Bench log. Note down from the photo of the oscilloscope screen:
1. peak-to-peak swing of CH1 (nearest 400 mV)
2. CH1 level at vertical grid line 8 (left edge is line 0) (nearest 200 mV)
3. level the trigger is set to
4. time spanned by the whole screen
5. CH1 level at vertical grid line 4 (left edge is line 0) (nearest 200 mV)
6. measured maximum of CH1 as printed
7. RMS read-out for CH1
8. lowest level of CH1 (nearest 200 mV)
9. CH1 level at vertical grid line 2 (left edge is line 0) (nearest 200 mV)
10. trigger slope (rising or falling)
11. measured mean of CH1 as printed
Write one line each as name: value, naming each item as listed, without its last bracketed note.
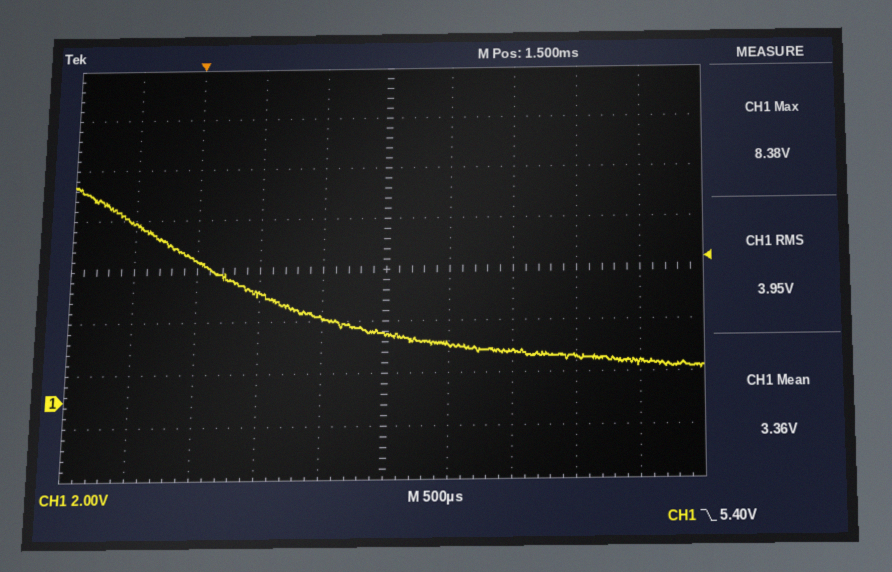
peak-to-peak swing of CH1: 7.2 V
CH1 level at vertical grid line 8 (left edge is line 0): 1.6 V
level the trigger is set to: 5.40 V
time spanned by the whole screen: 5 ms
CH1 level at vertical grid line 4 (left edge is line 0): 3.2 V
measured maximum of CH1 as printed: 8.38 V
RMS read-out for CH1: 3.95 V
lowest level of CH1: 1.2 V
CH1 level at vertical grid line 2 (left edge is line 0): 5.4 V
trigger slope: falling
measured mean of CH1 as printed: 3.36 V
